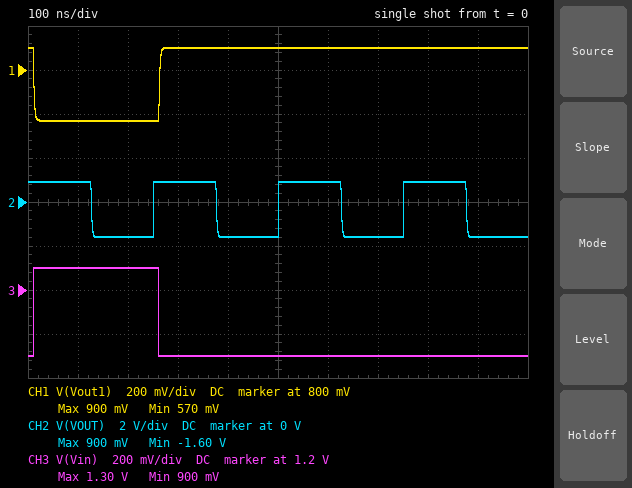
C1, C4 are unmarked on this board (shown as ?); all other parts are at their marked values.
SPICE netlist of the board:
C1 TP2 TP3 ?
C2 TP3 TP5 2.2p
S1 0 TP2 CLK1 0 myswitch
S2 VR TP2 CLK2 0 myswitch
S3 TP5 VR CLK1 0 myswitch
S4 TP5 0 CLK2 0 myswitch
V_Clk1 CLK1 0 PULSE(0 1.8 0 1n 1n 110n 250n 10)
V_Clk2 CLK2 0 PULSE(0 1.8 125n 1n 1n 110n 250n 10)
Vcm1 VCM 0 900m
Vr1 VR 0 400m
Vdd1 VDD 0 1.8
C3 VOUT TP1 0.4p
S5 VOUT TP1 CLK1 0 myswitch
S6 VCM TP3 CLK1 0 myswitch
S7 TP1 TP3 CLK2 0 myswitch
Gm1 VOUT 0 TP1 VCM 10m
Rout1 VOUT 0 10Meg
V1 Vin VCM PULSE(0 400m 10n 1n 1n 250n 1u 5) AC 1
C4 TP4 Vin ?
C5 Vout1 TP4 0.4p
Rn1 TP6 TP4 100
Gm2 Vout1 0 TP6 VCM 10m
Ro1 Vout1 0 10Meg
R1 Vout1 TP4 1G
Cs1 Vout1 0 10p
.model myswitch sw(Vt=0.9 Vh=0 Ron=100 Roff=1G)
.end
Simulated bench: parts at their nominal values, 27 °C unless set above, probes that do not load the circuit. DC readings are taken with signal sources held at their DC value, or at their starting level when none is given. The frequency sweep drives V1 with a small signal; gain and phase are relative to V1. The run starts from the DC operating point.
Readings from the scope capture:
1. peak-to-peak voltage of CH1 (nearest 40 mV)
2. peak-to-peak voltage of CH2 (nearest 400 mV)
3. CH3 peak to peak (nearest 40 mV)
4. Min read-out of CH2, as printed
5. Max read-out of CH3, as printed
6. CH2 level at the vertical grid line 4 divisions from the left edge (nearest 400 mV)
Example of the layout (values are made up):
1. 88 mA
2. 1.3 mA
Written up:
1. 320 mV
2. 2.4 V
3. 400 mV
4. -1.60 V
5. 1.30 V
6. -1.6 V
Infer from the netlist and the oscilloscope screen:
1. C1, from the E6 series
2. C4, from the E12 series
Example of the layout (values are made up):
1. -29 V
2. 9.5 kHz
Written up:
1. 4.7 pF
2. 330 fF
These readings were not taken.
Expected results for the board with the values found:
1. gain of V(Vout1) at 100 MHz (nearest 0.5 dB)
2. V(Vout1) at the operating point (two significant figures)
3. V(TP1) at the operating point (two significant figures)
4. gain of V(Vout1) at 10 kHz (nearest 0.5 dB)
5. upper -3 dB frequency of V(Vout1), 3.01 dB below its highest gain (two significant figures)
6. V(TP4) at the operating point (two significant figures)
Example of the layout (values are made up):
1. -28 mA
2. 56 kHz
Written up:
1. -5.5 dB
2. 900 mV
3. 900 mV
4. -1.5 dB
5. 86 MHz
6. 900 mV
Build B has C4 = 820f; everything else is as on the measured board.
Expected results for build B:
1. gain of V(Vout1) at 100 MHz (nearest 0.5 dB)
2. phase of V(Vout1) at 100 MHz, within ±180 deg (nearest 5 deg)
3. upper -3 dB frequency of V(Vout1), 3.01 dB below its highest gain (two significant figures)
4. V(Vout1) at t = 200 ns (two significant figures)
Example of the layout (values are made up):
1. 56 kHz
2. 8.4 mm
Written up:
1. -0.5 dB
2. 115 deg
3. 51 MHz
4. 80 mV
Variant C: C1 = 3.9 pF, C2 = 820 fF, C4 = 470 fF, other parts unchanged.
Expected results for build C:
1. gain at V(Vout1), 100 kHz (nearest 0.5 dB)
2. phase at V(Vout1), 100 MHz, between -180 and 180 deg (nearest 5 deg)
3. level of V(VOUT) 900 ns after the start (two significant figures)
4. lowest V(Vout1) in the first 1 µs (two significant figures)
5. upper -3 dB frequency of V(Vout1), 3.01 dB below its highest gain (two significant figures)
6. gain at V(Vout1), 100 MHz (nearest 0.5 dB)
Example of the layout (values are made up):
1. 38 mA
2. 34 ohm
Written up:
1. 1.5 dB
2. 125 deg
3. -2.2 V
4. 430 mV
5. 72 MHz
6. -3.5 dB
